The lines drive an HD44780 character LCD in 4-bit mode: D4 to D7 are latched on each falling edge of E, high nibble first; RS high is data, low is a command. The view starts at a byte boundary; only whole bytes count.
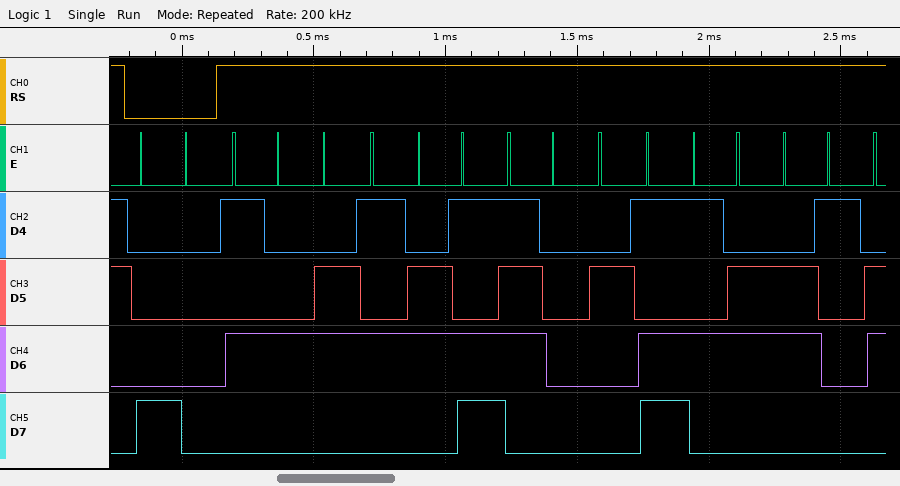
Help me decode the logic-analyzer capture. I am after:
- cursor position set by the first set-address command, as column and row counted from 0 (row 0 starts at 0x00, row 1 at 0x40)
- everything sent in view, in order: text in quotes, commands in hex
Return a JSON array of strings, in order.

["column 0, row 0", "0x80 \"Temp-Va\""]
